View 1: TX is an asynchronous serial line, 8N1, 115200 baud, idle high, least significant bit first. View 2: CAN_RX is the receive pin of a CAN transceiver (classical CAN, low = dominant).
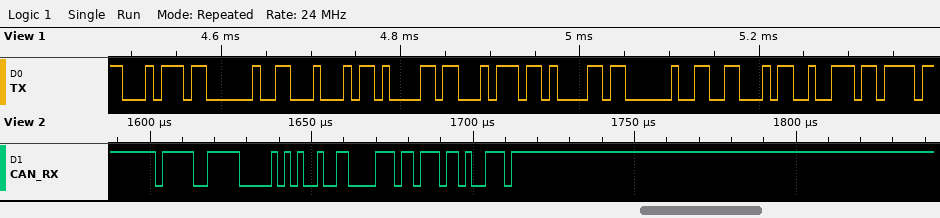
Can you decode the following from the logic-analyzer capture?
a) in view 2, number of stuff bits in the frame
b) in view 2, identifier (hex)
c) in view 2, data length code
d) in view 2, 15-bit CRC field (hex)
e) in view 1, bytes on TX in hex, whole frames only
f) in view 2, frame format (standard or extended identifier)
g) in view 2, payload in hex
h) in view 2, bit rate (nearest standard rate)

3
0x7DF
2
0x6ED3
0x74 0x20 0x44 0x61 0x74 0x61 0x20 0x46 0x72
standard
93 0E
500 kbit/s
